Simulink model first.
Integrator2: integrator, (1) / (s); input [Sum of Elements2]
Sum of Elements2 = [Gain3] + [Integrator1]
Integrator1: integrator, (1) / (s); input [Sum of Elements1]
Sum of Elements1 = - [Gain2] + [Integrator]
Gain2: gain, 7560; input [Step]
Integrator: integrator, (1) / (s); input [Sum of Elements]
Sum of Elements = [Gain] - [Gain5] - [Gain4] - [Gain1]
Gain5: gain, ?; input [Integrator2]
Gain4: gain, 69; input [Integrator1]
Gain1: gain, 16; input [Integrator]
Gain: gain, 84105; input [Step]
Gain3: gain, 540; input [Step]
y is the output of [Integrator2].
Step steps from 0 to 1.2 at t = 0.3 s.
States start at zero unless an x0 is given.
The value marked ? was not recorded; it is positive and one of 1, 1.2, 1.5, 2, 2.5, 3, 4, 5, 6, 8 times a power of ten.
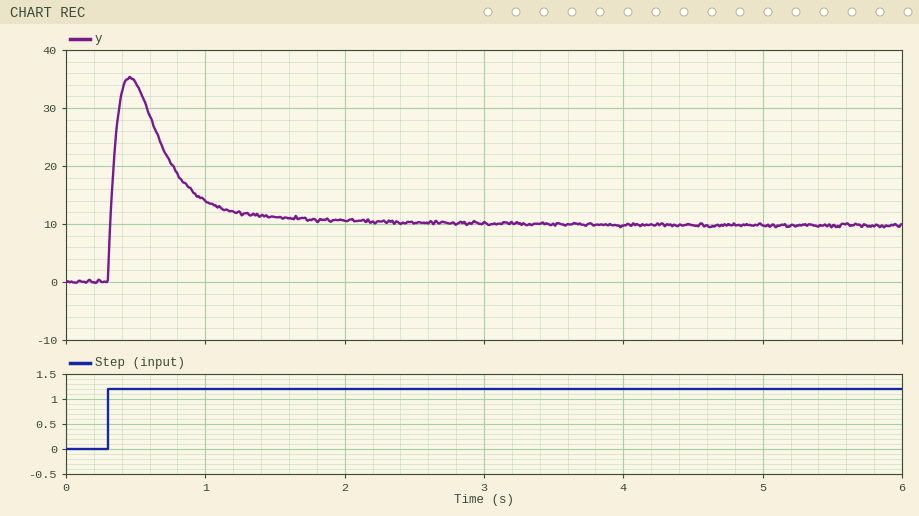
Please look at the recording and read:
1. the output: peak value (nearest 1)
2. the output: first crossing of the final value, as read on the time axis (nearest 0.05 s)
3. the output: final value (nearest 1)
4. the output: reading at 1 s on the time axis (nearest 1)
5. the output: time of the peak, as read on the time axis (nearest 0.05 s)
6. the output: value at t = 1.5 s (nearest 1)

35
0.30 s
10
14
0.45 s
11
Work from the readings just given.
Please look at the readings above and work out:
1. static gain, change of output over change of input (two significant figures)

8.3
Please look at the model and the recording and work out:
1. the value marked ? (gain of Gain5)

50
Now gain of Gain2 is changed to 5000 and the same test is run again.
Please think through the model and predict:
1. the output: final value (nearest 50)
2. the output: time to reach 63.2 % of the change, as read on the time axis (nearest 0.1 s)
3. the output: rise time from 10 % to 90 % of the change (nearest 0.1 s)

1000
1.6 s
2.5 s
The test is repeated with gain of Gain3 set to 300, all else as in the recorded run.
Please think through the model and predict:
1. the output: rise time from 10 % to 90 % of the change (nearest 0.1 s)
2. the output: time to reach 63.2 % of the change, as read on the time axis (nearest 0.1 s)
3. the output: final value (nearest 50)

2.4 s
1.5 s
-400
